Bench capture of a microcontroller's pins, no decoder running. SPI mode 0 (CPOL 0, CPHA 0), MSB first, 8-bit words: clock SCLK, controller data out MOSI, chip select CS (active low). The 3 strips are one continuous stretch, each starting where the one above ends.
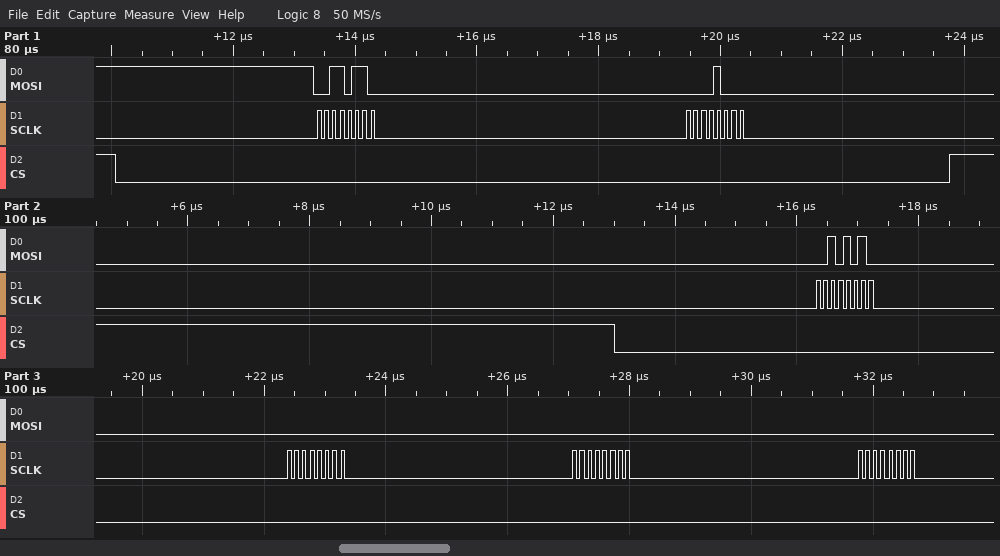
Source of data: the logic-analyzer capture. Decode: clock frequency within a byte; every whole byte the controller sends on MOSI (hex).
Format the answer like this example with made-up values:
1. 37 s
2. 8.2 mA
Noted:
1. 8 MHz
2. 36 08 2A 00 00 00
